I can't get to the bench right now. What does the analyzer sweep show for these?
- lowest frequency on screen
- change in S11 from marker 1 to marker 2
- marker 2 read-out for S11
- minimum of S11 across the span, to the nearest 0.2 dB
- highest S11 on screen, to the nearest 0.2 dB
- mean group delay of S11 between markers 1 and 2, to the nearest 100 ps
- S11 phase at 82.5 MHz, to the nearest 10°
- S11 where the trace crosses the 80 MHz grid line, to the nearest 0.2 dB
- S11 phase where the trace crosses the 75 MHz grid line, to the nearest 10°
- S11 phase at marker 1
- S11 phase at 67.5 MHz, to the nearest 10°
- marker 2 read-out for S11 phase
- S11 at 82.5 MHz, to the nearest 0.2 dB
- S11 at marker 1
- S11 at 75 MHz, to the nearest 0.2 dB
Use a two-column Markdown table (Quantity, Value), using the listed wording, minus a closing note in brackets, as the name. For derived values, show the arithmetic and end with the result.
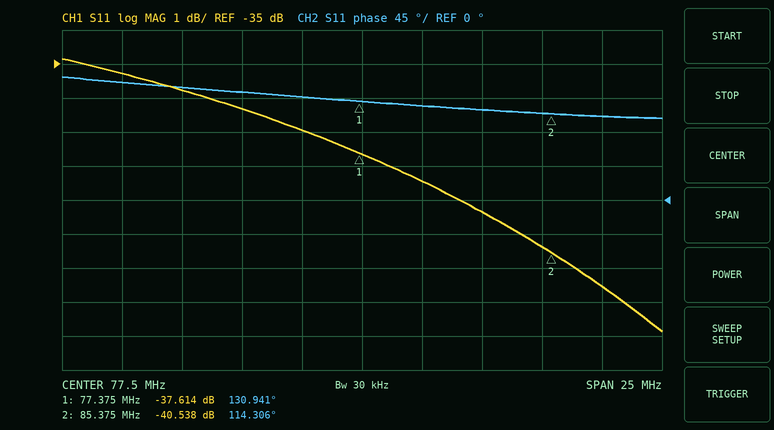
| Quantity | Value |
|---|---|
| lowest frequency on screen | 65 MHz |
| change in S11 from marker 1 to marker 2 | -40.538 − (-37.614) = -2.924 dB |
| marker 2 read-out for S11 | -40.538 dB |
| minimum of S11 across the span, to the nearest 0.2 dB | -42.8 dB |
| highest S11 on screen, to the nearest 0.2 dB | -34.8 dB |
| mean group delay of S11 between markers 1 and 2, to the nearest 100 ps | −(114.306° − (130.941°))/(360° × 8 MHz) ≈ 5.8 ns |
| S11 phase at 82.5 MHz, to the nearest 10° | 120° |
| S11 where the trace crosses the 80 MHz grid line, to the nearest 0.2 dB | -38.4 dB |
| S11 phase where the trace crosses the 75 MHz grid line, to the nearest 10° | 140° |
| S11 phase at marker 1 | 130.941° |
| S11 phase at 67.5 MHz, to the nearest 10° | 160° |
| marker 2 read-out for S11 phase | 114.306° |
| S11 at 82.5 MHz, to the nearest 0.2 dB | -39.4 dB |
| S11 at marker 1 | -37.614 dB |
| S11 at 75 MHz, to the nearest 0.2 dB | -37.0 dB |
